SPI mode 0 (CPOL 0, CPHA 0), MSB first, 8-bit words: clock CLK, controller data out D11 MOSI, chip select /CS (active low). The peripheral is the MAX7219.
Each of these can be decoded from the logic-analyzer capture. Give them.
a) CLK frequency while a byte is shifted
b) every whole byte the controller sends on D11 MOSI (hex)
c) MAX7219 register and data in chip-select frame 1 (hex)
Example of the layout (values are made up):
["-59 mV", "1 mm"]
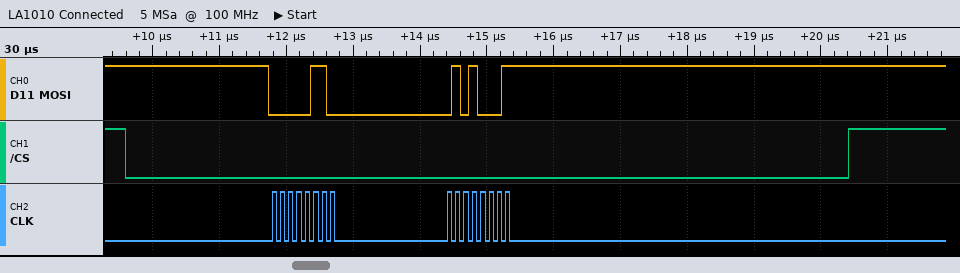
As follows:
["8 MHz", "06 51", "register 0x6, data 0x51"]
